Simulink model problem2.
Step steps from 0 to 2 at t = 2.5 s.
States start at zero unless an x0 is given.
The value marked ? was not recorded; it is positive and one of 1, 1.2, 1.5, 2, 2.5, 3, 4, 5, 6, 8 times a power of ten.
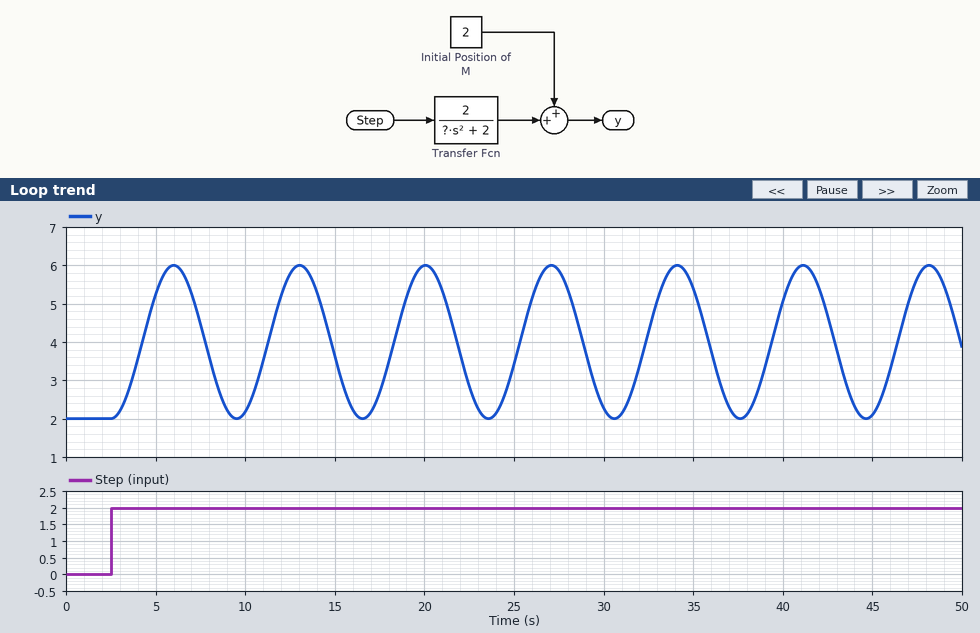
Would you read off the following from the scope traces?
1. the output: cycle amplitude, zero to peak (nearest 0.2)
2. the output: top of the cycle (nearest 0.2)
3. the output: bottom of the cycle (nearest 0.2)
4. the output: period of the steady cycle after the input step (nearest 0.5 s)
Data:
2.0
6.0
2.0
7.0 s
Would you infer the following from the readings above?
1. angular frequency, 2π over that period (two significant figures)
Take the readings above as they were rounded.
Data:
0.90 rad/s
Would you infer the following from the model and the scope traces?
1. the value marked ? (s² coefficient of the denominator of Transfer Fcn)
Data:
2.5
